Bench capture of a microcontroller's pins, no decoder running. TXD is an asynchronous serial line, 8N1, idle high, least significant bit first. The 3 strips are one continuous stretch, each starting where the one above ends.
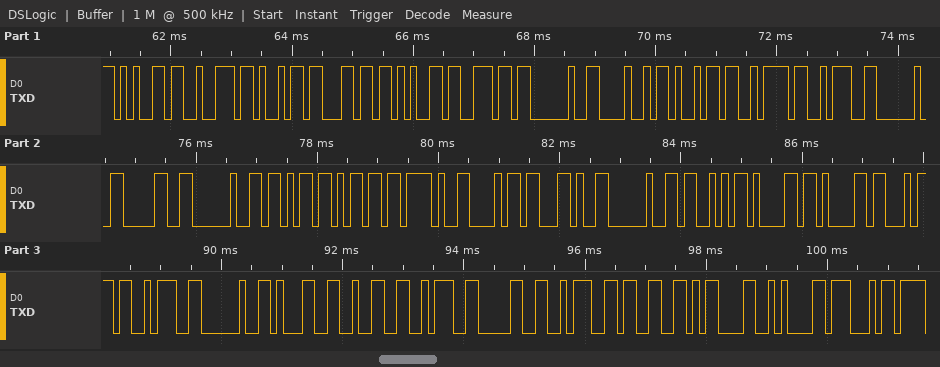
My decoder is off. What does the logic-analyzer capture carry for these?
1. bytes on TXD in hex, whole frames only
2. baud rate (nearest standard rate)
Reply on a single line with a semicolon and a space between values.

0x65 0x72 0x69 0x6C 0x65 0x6E 0x20 0x48 0x69 0x7A 0x3A 0x20 0x30 0x20 0x6B 0x6D 0x2F 0x68 0x2C 0x20 0x53 0x61 0x61 0x74 0x3A 0x20 0x31 0x32 0x3A 0x30 0x3A 0x33 0x0D 0x0A 0x47; 9600 baud
